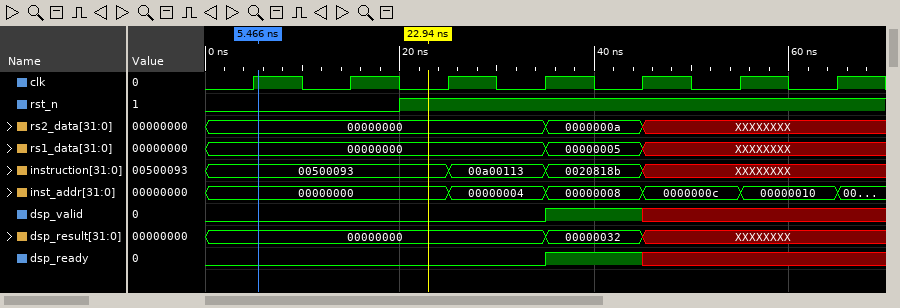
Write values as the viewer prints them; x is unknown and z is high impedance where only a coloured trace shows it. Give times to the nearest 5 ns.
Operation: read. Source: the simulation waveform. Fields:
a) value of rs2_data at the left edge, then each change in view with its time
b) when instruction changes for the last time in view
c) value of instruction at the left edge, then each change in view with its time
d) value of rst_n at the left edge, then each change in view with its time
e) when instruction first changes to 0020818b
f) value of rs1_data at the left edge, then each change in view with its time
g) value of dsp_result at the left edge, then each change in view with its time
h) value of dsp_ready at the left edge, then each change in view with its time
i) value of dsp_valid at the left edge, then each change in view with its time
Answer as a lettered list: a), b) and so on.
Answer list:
a) 00000000, 0000000a at 35 ns, XXXXXXXX at 45 ns
b) 45 ns
c) 00500093, 00a00113 at 25 ns, 0020818b at 35 ns, XXXXXXXX at 45 ns
d) 0, 1 at 20 ns
e) 35 ns
f) 00000000, 00000005 at 35 ns, XXXXXXXX at 45 ns
g) 00000000, 00000032 at 35 ns, XXXXXXXX at 45 ns
h) 0, 1 at 35 ns, x at 45 ns
i) 0, 1 at 35 ns, x at 45 ns
